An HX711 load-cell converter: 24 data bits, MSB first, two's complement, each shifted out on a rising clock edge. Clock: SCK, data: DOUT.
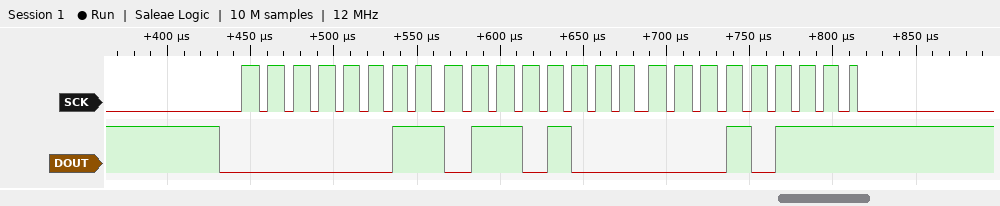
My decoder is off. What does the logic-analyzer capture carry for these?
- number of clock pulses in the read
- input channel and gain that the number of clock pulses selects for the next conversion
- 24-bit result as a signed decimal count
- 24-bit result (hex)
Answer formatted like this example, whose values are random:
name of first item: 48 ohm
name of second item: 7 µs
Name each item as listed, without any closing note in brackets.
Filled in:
number of clock pulses in the read: 25
input channel and gain that the number of clock pulses selects for the next conversion: channel A, gain 128
24-bit result as a signed decimal count: 223255
24-bit result: 0x036817
